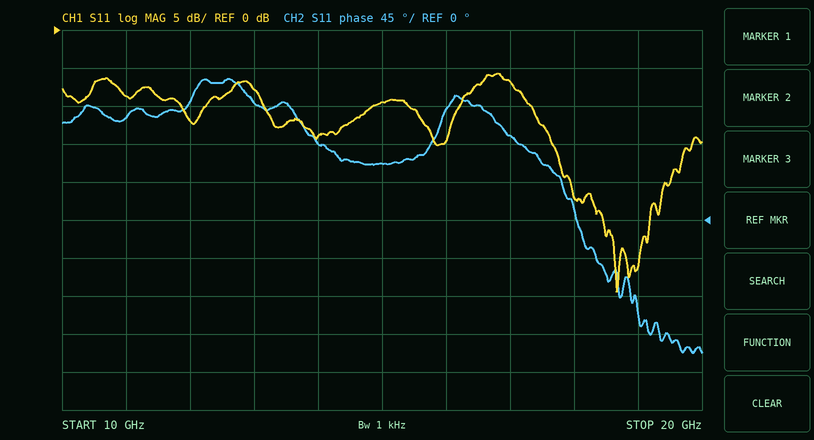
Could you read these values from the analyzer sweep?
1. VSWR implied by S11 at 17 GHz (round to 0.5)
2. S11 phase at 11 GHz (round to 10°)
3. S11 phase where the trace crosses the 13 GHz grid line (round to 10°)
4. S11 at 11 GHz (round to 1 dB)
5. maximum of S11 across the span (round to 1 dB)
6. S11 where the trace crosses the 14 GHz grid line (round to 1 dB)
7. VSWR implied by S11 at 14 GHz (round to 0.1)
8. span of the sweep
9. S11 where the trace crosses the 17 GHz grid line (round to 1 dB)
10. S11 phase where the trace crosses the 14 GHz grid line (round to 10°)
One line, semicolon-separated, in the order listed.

2.5; 120°; 140°; -9 dB; -6 dB; -14 dB; 1.5; 10 GHz; -7 dB; 90°
